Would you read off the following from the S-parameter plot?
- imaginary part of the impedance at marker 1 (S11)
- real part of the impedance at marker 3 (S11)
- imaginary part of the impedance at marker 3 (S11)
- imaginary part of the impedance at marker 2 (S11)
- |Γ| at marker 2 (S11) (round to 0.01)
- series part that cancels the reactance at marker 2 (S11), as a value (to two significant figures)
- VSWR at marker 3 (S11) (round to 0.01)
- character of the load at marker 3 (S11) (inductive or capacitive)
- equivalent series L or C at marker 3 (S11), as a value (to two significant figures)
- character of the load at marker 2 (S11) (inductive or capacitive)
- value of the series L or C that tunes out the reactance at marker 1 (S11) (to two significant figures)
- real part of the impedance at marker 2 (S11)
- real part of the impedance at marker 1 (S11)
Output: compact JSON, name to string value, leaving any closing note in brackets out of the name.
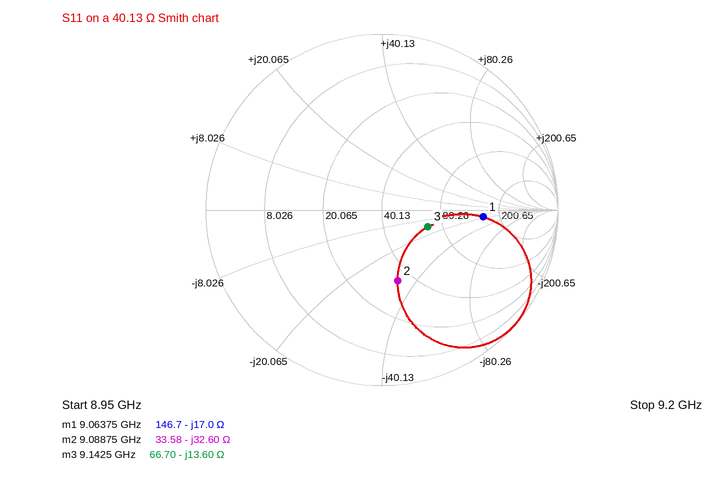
{"imaginary part of the impedance at marker 1": "-17.0 Ω", "real part of the impedance at marker 3": "66.70 Ω", "imaginary part of the impedance at marker 3": "-13.60 Ω", "imaginary part of the impedance at marker 2": "-32.60 Ω", "|Γ| at marker 2 (S11)": "0.41", "series part that cancels the reactance at marker 2 (S11), as a value": "570 pH", "VSWR at marker 3 (S11)": "1.77", "character of the load at marker 3 (S11)": "capacitive", "equivalent series L or C at marker 3 (S11), as a value": "1.3 pF", "character of the load at marker 2 (S11)": "capacitive", "value of the series L or C that tunes out the reactance at marker 1 (S11)": "300 pH", "real part of the impedance at marker 2": "33.58 Ω", "real part of the impedance at marker 1": "146.7 Ω"}
